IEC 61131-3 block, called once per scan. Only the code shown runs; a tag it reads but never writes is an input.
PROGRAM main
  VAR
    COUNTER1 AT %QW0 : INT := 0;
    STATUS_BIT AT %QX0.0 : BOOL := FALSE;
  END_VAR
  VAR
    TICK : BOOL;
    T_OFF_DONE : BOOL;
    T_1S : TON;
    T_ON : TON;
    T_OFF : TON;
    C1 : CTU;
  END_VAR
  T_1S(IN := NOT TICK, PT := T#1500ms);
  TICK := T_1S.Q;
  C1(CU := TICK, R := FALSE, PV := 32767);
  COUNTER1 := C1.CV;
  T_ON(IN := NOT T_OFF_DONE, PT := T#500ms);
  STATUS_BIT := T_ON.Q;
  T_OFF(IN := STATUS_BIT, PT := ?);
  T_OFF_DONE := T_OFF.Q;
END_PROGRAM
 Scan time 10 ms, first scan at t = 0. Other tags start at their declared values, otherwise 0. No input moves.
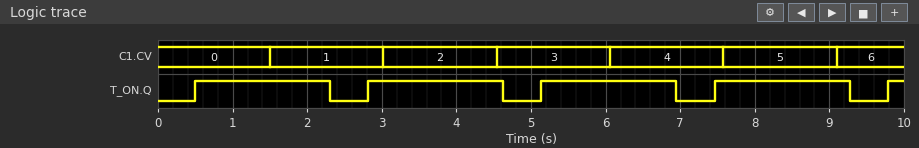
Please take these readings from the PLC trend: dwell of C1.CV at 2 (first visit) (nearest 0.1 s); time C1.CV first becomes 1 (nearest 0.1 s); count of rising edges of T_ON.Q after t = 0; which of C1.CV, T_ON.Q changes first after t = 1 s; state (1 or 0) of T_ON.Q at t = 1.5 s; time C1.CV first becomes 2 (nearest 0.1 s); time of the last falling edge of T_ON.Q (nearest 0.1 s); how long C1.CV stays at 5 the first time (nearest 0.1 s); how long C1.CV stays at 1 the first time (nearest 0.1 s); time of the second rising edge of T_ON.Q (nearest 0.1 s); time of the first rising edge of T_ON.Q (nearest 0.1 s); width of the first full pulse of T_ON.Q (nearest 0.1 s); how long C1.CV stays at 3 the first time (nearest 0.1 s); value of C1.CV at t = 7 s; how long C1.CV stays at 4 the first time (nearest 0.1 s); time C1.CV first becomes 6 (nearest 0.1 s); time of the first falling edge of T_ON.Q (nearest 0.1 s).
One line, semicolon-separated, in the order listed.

1.5 s; 1.5 s; 5; C1.CV; 1; 3.0 s; 9.3 s; 1.5 s; 1.5 s; 2.8 s; 0.5 s; 1.8 s; 1.5 s; 4; 1.5 s; 9.1 s; 2.3 s
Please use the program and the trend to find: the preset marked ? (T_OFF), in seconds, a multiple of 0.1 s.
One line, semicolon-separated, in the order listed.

1.8 s
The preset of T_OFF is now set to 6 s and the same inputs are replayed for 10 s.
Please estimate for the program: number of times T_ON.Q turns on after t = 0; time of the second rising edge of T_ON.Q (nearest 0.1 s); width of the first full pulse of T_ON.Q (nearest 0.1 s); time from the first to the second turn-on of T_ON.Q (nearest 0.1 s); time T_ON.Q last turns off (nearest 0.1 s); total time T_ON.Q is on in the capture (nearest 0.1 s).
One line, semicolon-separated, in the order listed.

2; 7.0 s; 6.0 s; 6.5 s; 6.5 s; 9.0 s
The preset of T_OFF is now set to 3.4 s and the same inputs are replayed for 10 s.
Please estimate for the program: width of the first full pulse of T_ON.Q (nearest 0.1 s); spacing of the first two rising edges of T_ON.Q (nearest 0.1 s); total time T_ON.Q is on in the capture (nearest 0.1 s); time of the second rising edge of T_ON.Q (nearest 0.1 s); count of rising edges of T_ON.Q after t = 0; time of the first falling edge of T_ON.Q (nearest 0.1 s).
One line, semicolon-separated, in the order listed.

3.4 s; 3.9 s; 8.5 s; 4.4 s; 3; 3.9 s
